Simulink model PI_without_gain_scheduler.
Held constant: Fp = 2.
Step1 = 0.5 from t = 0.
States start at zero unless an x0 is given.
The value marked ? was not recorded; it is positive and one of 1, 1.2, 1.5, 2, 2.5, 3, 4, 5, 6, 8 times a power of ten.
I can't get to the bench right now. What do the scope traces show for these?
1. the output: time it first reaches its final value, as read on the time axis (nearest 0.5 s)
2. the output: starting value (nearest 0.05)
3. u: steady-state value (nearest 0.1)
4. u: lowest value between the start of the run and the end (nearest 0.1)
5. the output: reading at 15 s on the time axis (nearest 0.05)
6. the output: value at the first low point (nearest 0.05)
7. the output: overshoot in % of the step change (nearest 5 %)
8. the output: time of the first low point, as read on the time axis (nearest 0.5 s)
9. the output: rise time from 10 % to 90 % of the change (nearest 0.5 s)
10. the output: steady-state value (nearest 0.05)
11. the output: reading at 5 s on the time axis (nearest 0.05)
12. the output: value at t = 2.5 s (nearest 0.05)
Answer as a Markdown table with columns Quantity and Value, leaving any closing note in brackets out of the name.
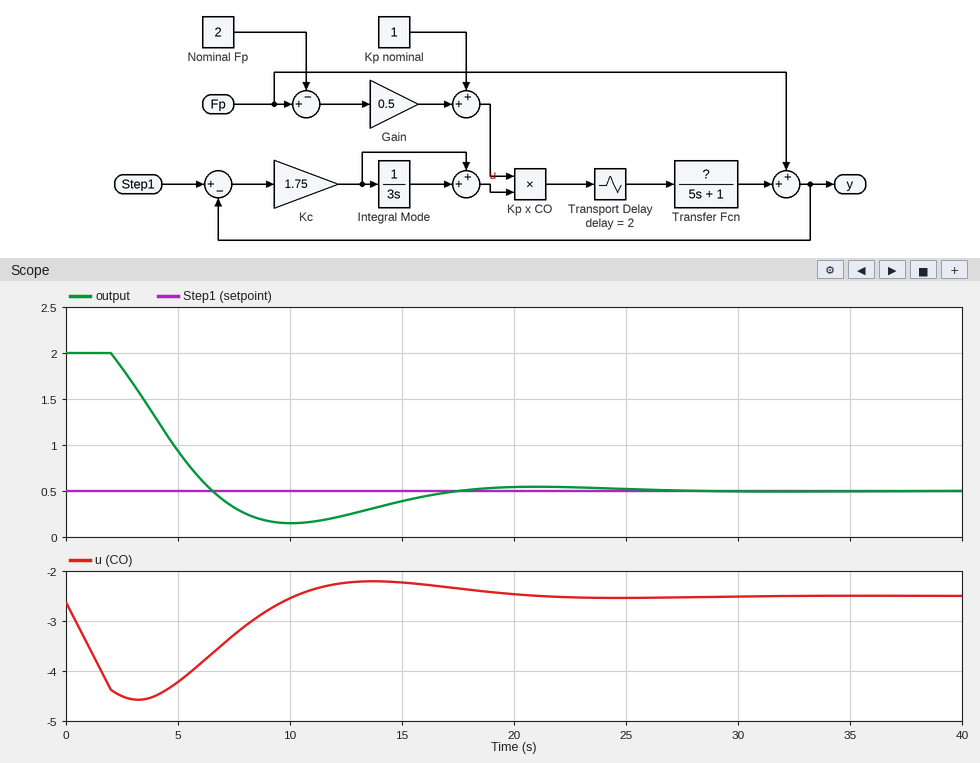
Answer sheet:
| Quantity | Value |
|---|---|
| the output: time it first reaches its final value, as read on the time axis | 6.5 s |
| the output: starting value | 2.00 |
| u: steady-state value | -2.5 |
| u: lowest value between the start of the run and the end | -4.6 |
| the output: reading at 15 s on the time axis | 0.40 |
| the output: value at the first low point | 0.15 |
| the output: overshoot in % of the step change | 25 % |
| the output: time of the first low point, as read on the time axis | 10.0 s |
| the output: rise time from 10 % to 90 % of the change | 3.5 s |
| the output: steady-state value | 0.50 |
| the output: reading at 5 s on the time axis | 0.95 |
| the output: value at t = 2.5 s | 1.85 |
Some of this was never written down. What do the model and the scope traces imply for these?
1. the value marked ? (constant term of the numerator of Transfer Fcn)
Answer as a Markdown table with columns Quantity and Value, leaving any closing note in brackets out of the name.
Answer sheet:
| Quantity | Value |
|---|---|
| the value marked ? | 0.6 |
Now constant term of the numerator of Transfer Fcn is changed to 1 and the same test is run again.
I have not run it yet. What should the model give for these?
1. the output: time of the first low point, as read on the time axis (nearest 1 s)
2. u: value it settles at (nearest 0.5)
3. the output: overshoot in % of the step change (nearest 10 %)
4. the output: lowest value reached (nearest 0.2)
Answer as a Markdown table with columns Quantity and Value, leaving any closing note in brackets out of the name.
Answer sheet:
| Quantity | Value |
|---|---|
| the output: time of the first low point, as read on the time axis | 7 s |
| u: value it settles at | -1.5 |
| the output: overshoot in % of the step change | 50 % |
| the output: lowest value reached | -0.2 |
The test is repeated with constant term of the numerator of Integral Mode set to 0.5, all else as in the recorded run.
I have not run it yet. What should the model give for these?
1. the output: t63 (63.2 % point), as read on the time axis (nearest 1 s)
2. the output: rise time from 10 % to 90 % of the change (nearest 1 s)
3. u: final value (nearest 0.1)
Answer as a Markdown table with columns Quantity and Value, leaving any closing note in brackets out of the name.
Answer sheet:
| Quantity | Value |
|---|---|
| the output: t63 (63.2 % point), as read on the time axis | 5 s |
| the output: rise time from 10 % to 90 % of the change | 7 s |
| u: final value | -2.5 |
